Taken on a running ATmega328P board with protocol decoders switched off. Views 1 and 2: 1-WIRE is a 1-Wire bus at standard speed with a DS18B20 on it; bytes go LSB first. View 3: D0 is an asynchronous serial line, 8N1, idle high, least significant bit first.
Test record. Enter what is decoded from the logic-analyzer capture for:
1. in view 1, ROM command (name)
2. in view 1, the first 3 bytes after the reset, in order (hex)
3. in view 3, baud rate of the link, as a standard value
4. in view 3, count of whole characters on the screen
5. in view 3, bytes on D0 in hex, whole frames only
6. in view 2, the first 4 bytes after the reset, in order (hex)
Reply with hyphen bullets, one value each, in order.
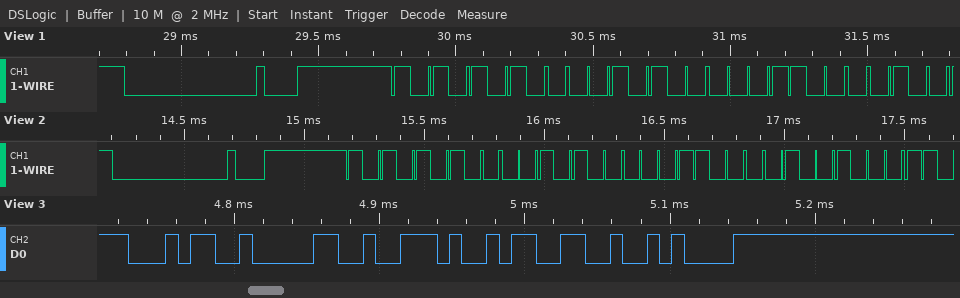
- Match ROM
- 55 28 18
- 115200 baud
- 5
- 0x34 0x30 0x2E 0x33 0x0A
- 55 28 18 12
